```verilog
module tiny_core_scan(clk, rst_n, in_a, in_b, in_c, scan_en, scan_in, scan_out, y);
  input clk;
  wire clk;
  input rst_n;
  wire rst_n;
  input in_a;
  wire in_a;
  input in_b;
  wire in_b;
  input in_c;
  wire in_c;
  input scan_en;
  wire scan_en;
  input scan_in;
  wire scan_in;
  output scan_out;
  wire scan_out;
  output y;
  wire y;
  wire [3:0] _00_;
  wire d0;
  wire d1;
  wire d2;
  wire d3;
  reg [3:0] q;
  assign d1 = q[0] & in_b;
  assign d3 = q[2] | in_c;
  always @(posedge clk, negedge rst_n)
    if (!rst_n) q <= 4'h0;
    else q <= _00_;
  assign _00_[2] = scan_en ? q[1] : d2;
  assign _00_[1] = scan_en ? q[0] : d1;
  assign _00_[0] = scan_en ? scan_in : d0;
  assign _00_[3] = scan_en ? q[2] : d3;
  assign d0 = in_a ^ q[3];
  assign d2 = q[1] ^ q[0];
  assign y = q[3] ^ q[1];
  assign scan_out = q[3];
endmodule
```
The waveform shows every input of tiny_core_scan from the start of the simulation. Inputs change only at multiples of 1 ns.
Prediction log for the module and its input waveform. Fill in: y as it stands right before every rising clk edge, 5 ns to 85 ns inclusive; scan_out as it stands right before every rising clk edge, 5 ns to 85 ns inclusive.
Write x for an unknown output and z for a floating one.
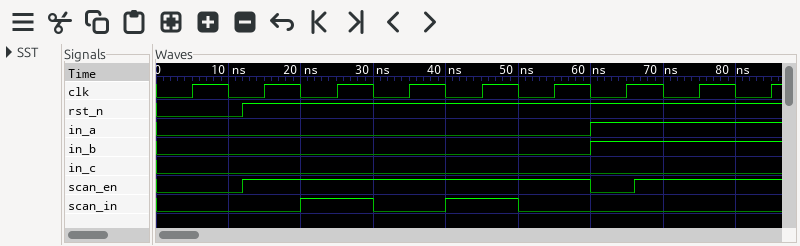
0 0 0 0 1 0 0 0 1
0 0 0 0 0 0 1 0 1
